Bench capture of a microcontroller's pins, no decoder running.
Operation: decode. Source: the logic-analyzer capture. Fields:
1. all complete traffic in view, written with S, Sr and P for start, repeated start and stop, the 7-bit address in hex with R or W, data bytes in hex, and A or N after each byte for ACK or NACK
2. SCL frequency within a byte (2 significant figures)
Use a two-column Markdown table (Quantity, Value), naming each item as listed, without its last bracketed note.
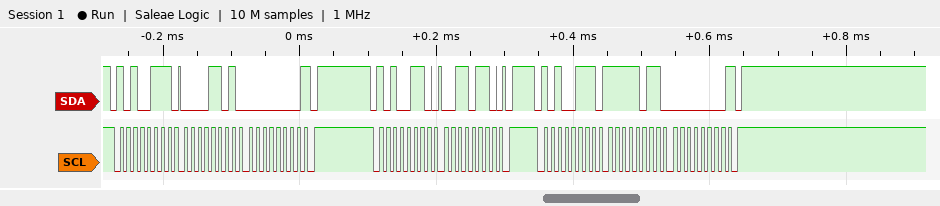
| Quantity | Value |
|---|---|
| all complete traffic in view, written with S, Sr and P for start, repeated start and stop, the 7-bit address in hex with R or W, data bytes in hex, and A or N after each byte for ACK or NACK | S 53R A 0D A 00 N P S 53W A 36 A P S 53R A FB A 00 N P |
| SCL frequency within a byte | 100 kHz |
